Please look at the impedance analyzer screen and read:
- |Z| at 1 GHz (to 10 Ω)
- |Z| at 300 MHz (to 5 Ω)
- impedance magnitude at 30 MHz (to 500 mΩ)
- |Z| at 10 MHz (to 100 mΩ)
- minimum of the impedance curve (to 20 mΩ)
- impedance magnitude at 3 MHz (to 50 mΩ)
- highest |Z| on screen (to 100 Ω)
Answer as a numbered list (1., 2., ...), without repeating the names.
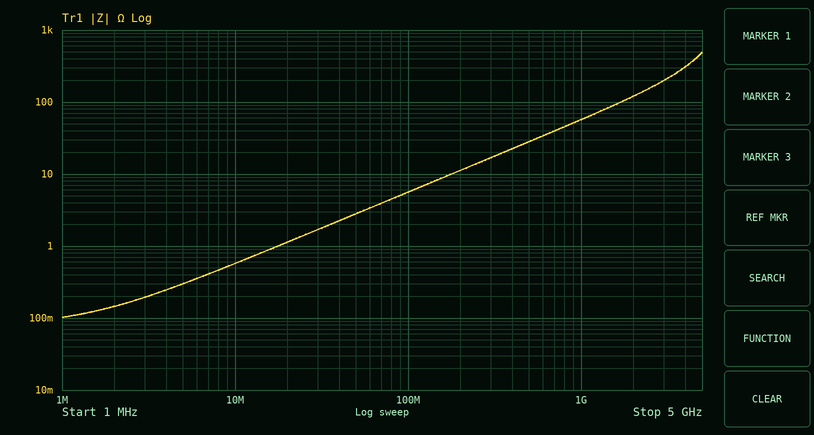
1. 60 Ω
2. 15 Ω
3. 1.5 Ω
4. 600 mΩ
5. 100 mΩ
6. 200 mΩ
7. 500 Ω
